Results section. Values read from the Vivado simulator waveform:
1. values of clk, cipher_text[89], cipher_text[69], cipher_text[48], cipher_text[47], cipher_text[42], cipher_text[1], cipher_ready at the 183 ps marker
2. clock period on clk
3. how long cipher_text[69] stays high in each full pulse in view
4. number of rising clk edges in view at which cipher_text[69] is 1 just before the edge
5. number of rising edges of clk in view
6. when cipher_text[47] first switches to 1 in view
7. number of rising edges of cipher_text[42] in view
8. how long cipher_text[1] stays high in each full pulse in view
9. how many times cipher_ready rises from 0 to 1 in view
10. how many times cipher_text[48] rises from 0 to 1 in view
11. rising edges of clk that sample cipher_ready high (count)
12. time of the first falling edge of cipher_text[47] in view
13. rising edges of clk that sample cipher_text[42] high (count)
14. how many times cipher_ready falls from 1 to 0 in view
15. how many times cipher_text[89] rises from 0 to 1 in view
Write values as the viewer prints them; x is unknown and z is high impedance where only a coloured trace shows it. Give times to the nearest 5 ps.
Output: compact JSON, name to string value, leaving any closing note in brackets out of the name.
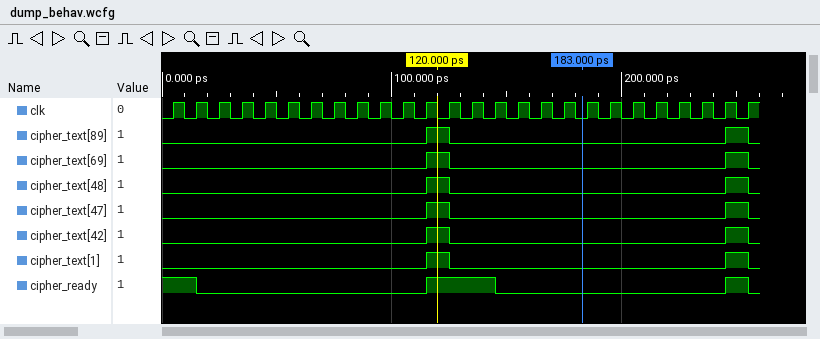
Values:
{"values of clk, cipher_text[89], cipher_text[69], cipher_text[48], cipher_text[47], cipher_text[42], cipher_text[1], cipher_ready at the 183 ps marker": "clk=0, cipher_text[89]=0, cipher_text[69]=0, cipher_text[48]=0, cipher_text[47]=0, cipher_text[42]=0, cipher_text[1]=0, cipher_ready=0", "clock period on clk": "10 ps", "how long cipher_text[69] stays high in each full pulse in view": "10 ps, 10 ps", "number of rising clk edges in view at which cipher_text[69] is 1 just before the edge": "2", "number of rising edges of clk in view": "26", "when cipher_text[47] first switches to 1 in view": "115 ps", "number of rising edges of cipher_text[42] in view": "2", "how long cipher_text[1] stays high in each full pulse in view": "10 ps, 10 ps", "how many times cipher_ready rises from 0 to 1 in view": "2", "how many times cipher_text[48] rises from 0 to 1 in view": "2", "rising edges of clk that sample cipher_ready high": "6", "time of the first falling edge of cipher_text[47] in view": "125 ps", "rising edges of clk that sample cipher_text[42] high": "2", "how many times cipher_ready falls from 1 to 0 in view": "3", "how many times cipher_text[89] rises from 0 to 1 in view": "2"}
